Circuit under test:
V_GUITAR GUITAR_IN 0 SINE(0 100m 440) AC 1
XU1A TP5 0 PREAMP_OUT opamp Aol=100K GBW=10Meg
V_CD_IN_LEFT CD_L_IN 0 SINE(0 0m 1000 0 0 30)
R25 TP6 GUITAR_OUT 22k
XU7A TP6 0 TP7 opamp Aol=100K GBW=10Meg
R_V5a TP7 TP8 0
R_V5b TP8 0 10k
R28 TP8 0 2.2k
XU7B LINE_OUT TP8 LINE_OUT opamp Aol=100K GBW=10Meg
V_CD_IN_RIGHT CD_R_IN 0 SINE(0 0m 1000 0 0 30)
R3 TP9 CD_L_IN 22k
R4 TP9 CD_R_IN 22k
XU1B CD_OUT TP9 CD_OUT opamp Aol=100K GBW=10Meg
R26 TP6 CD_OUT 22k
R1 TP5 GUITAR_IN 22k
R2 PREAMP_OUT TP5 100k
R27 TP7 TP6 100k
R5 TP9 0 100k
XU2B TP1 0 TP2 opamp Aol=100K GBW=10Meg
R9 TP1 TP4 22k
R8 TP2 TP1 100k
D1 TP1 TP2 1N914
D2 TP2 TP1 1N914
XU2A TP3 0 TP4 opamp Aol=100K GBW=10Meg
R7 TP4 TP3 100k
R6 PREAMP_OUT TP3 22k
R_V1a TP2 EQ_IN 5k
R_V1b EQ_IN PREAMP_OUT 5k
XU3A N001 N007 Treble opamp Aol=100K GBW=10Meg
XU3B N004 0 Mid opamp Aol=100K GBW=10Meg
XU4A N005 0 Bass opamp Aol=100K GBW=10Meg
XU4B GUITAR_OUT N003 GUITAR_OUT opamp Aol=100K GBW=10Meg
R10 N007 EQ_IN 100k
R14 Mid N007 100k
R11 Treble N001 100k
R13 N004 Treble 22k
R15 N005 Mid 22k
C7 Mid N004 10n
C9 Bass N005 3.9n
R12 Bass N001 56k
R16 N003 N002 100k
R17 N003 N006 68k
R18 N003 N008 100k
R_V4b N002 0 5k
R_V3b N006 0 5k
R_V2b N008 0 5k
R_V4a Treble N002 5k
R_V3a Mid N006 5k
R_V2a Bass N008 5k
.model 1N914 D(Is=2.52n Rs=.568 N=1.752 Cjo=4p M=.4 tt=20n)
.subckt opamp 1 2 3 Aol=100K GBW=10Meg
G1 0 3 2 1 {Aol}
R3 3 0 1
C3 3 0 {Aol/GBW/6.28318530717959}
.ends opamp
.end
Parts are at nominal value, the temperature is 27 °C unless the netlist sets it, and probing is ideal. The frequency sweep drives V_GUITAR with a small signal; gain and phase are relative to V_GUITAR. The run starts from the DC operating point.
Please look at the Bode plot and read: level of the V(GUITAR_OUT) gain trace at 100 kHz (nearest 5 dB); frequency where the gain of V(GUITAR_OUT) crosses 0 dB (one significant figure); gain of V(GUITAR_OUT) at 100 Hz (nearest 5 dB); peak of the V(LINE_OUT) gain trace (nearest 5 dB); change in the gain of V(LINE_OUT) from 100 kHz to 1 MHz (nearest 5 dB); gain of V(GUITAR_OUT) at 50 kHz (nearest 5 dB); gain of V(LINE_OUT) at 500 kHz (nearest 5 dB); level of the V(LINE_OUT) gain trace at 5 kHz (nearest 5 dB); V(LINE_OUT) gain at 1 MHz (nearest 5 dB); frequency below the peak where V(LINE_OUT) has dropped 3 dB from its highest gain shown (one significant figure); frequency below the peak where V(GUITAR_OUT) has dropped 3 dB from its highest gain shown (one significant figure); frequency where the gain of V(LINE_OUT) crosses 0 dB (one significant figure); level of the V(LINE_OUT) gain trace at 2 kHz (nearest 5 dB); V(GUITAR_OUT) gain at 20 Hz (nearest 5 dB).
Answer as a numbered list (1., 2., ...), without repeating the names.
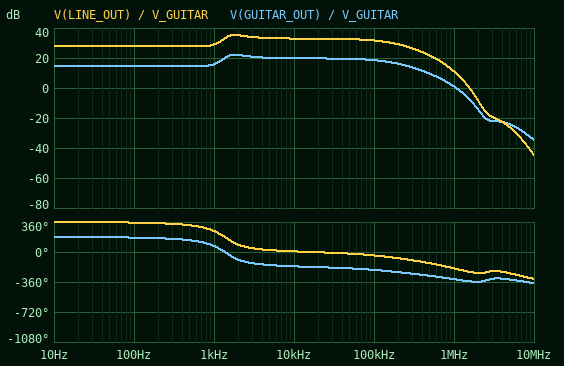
1. 20 dB
2. 1 MHz
3. 15 dB
4. 35 dB
5. -20 dB
6. 20 dB
7. 20 dB
8. 35 dB
9. 10 dB
10. 1 kHz
11. 1 kHz
12. 2 MHz
13. 35 dB
14. 15 dB
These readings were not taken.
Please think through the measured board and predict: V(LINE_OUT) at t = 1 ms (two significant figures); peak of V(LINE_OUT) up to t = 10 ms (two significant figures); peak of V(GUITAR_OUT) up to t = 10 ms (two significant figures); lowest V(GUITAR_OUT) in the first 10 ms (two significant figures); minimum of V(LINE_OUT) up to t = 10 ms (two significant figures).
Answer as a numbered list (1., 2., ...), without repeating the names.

1. 200 mV
2. 290 mV
3. 64 mV
4. -64 mV
5. -290 mV
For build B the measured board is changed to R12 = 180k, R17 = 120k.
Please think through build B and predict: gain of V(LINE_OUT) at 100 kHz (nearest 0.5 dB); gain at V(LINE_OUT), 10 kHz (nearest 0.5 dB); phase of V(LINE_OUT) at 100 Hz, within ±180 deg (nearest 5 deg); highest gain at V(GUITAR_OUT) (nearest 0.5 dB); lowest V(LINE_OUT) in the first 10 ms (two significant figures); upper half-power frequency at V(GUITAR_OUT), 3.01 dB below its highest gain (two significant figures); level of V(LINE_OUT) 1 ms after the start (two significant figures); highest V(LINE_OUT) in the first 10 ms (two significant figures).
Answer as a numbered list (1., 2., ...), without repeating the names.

1. 28.5 dB
2. 29.5 dB
3. -5 deg
4. 22.5 dB
5. -650 mV
6. 910 Hz
7. 530 mV
8. 640 mV
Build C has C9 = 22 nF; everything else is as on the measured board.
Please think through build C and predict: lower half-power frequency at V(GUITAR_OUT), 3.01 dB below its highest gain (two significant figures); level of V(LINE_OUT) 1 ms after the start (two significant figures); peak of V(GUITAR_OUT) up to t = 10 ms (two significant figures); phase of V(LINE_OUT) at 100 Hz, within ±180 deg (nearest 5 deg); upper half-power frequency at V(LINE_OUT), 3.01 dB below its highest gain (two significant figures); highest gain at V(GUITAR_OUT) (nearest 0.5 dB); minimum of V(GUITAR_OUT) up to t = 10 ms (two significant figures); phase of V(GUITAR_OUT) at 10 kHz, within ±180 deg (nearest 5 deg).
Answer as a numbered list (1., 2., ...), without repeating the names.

1. 320 Hz
2. 130 mV
3. 110 mV
4. -40 deg
5. 140 kHz
6. 20.5 dB
7. -110 mV
8. -170 deg
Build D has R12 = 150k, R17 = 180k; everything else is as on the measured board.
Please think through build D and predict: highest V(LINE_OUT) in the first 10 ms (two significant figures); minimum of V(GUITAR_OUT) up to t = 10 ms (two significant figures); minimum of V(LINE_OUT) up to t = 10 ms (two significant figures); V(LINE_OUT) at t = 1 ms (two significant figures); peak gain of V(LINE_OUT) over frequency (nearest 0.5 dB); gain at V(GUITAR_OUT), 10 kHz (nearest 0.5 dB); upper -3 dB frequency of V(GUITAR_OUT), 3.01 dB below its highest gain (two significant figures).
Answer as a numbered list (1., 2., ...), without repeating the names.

1. 610 mV
2. -130 mV
3. -610 mV
4. 480 mV
5. 35.0 dB
6. 18.0 dB
7. 920 Hz
